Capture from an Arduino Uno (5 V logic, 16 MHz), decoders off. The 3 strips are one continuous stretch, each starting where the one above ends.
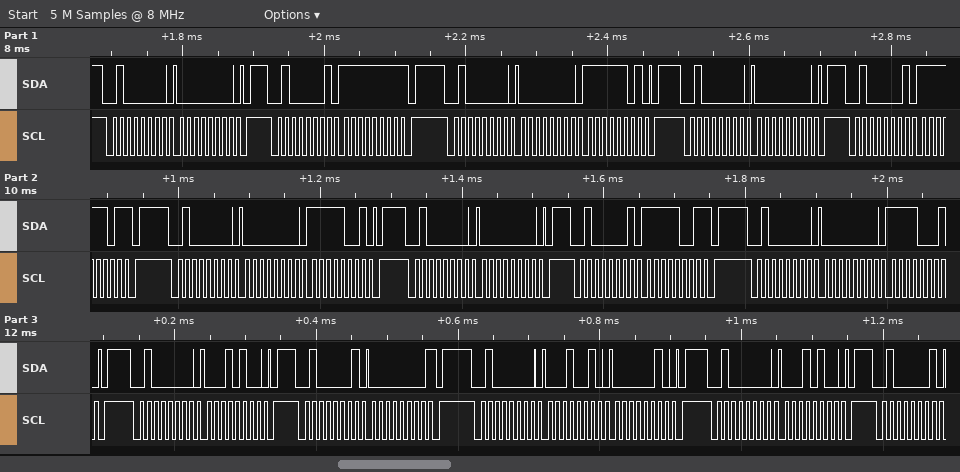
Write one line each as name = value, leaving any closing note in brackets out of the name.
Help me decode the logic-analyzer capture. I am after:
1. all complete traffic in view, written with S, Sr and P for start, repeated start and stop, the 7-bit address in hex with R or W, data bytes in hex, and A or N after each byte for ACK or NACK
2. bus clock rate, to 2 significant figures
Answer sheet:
all complete traffic in view, written with S, Sr and P for start, repeated start and stop, the 7-bit address in hex with R or W, data bytes in hex, and A or N after each byte for ACK or NACK = S 20W A 00 A P S 20R A FF N P S 20W A 00 A FD A P S 20W A 00 A P S 20R A FD N P S 20W A 00 A F9 A P S 20W A 00 A P S 20R A F9 N P S 20W A 00 A F1 A P S 20W A 14 A P S 20R A 00 N P S 20W A 12 A 02 A P S 20W A 14 A P S 20R A
bus clock rate, to 2 significant figures = 100 kHz
